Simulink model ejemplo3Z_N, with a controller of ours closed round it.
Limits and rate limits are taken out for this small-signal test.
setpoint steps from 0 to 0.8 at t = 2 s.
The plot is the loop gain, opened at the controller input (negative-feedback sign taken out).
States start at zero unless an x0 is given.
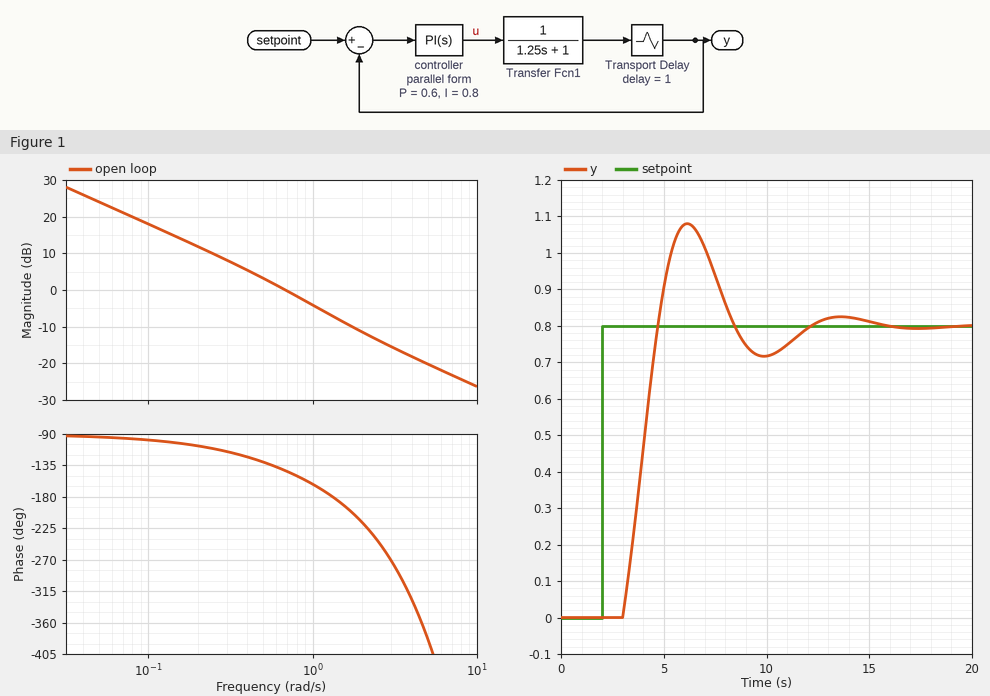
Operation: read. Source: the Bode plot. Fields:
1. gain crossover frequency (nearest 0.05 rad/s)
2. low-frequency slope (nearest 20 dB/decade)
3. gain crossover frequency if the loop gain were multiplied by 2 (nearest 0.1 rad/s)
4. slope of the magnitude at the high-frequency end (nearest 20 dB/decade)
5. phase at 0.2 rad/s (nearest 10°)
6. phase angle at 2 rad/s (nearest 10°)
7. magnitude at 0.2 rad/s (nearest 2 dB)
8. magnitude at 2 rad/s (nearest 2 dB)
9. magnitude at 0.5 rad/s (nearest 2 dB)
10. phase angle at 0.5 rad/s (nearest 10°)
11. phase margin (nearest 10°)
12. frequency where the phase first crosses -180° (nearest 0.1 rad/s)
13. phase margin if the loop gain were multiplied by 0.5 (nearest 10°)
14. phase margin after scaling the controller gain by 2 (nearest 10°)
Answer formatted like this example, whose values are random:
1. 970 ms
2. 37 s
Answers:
1. 0.70 rad/s
2. -20 dB/decade
3. 1.2 rad/s
4. -20 dB/decade
5. -110°
6. -220°
7. 12 dB
8. -12 dB
9. 4 dB
10. -130°
11. 40°
12. 1.3 rad/s
13. 60°
14. 10°
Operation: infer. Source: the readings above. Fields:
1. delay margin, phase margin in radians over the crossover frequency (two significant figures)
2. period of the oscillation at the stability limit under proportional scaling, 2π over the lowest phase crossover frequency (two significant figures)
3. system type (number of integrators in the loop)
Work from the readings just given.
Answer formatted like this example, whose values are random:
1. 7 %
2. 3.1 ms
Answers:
1. 1.00 s
2. 4.8 s
3. 1
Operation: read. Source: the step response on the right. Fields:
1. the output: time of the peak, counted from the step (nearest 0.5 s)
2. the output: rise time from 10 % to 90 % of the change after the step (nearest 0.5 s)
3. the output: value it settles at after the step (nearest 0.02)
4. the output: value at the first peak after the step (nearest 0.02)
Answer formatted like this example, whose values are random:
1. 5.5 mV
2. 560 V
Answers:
1. 4.0 s
2. 1.5 s
3. 0.80
4. 1.08
